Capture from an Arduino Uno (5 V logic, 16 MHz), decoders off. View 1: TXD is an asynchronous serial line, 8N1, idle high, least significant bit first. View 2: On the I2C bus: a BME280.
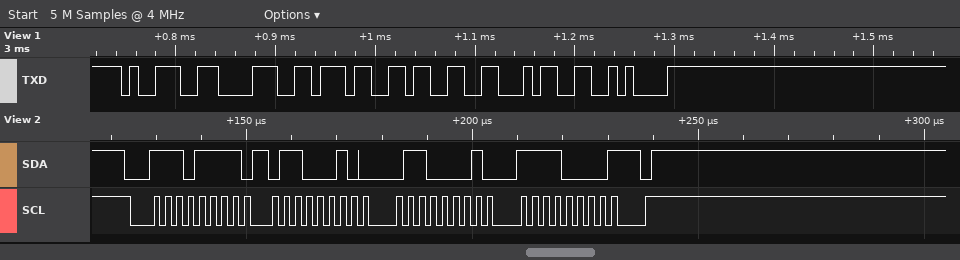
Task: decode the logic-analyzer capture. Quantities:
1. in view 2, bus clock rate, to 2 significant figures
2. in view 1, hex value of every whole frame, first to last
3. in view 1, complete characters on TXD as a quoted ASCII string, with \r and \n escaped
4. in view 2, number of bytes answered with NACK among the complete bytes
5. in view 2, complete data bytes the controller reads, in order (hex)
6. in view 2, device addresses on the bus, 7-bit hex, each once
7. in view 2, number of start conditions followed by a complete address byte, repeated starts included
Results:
400 kHz
39 38 37 33 34 0A
"98734\n"
1
62 61 F0
0x77
1
